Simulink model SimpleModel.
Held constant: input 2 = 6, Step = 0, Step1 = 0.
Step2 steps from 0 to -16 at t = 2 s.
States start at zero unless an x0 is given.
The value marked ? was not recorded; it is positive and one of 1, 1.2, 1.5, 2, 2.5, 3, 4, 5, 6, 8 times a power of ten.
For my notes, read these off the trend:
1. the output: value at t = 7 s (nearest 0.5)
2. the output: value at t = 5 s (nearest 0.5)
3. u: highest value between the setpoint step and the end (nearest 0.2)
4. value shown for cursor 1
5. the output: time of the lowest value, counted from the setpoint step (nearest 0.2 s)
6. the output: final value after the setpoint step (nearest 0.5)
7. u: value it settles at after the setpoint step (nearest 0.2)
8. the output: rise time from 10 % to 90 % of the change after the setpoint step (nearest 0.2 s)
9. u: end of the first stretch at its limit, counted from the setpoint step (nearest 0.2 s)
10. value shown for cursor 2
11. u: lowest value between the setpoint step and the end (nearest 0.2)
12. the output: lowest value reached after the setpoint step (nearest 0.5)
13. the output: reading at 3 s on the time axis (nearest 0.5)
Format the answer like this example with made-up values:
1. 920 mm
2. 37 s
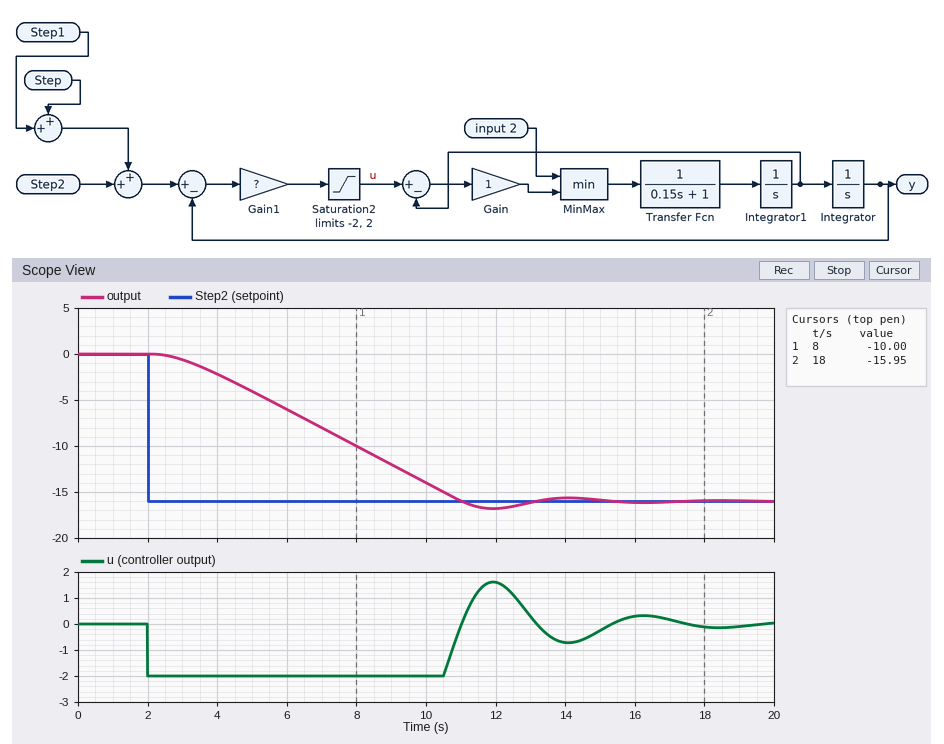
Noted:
1. -8.0
2. -4.0
3. 1.6
4. -10.00
5. 10.0 s
6. -16.0
7. 0.0
8. 6.6 s
9. 8.6 s
10. -15.95
11. -2.0
12. -17.0
13. -0.5
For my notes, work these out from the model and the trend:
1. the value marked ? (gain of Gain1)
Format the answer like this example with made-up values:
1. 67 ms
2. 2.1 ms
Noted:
1. 2
